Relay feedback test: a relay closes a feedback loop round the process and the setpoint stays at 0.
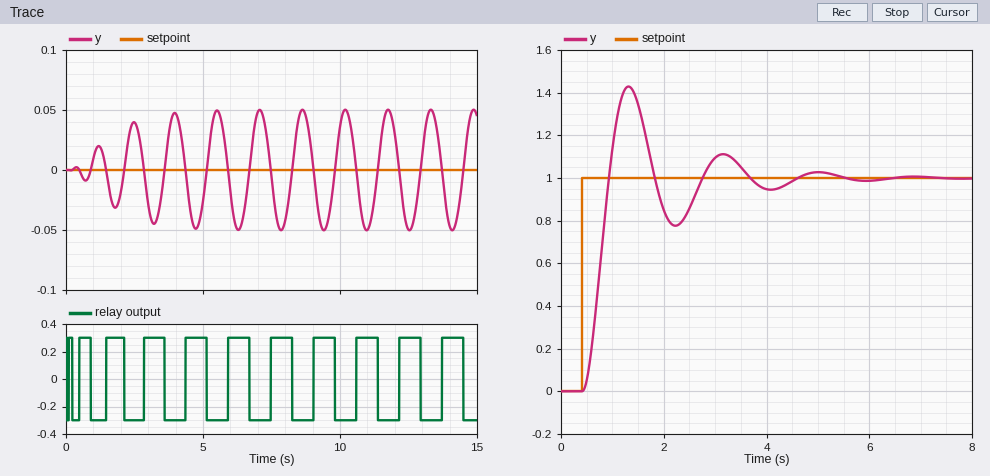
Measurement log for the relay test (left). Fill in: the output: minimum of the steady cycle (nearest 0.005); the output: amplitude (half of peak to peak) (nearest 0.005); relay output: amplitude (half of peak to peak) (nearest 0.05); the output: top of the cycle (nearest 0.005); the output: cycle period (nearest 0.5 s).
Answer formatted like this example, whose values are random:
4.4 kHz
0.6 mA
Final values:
-0.050
0.050
0.30
0.050
1.5 s
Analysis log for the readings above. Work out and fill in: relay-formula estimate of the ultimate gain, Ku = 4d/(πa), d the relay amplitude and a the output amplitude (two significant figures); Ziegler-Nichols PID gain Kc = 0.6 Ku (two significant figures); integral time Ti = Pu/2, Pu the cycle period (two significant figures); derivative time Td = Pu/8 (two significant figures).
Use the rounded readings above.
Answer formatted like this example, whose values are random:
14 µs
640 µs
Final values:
7.6
4.6
0.75 s
0.19 s
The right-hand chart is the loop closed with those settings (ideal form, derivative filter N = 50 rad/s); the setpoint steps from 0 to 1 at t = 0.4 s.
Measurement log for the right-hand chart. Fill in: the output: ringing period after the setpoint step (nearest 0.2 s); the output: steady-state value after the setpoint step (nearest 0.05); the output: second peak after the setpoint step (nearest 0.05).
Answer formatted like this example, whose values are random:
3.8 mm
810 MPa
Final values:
1.8 s
1.00
1.10
